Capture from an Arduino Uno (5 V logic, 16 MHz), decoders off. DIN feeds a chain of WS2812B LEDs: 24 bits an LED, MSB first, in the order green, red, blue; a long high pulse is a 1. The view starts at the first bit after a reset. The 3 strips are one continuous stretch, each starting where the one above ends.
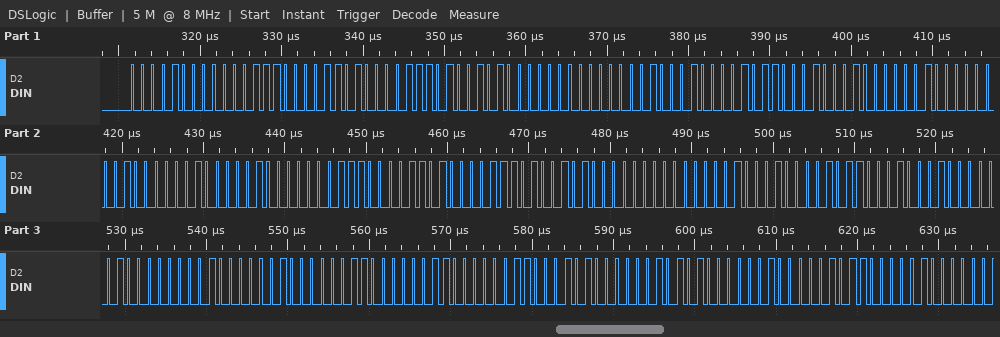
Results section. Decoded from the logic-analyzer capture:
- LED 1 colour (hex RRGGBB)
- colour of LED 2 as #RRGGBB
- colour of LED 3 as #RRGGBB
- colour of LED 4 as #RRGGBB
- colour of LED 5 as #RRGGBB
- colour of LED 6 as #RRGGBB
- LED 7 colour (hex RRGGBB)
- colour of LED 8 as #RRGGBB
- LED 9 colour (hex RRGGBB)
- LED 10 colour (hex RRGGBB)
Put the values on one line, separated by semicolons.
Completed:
#0E081A; #281D00; #0B1111; #010202; #0E081A; #281D00; #0B1111; #010202; #060606; #152802
